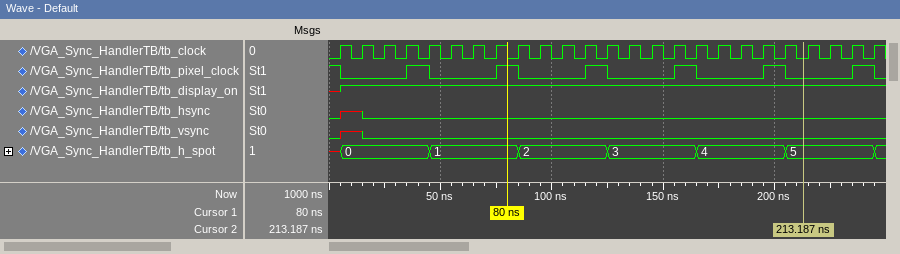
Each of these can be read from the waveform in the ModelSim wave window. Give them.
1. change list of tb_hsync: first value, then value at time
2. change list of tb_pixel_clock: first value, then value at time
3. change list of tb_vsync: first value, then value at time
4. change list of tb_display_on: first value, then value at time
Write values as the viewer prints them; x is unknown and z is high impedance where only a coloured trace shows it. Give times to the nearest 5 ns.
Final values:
0, x at 5 ns, 0 at 15 ns
1, 0 at 5 ns, 1 at 35 ns, 0 at 45 ns, 1 at 75 ns, 0 at 85 ns, 1 at 115 ns, 0 at 125 ns, 1 at 155 ns, 0 at 165 ns, 1 at 195 ns, 0 at 205 ns, 1 at 235 ns, 0 at 245 ns
0, x at 5 ns, 0 at 15 ns
x, 1 at 5 ns
